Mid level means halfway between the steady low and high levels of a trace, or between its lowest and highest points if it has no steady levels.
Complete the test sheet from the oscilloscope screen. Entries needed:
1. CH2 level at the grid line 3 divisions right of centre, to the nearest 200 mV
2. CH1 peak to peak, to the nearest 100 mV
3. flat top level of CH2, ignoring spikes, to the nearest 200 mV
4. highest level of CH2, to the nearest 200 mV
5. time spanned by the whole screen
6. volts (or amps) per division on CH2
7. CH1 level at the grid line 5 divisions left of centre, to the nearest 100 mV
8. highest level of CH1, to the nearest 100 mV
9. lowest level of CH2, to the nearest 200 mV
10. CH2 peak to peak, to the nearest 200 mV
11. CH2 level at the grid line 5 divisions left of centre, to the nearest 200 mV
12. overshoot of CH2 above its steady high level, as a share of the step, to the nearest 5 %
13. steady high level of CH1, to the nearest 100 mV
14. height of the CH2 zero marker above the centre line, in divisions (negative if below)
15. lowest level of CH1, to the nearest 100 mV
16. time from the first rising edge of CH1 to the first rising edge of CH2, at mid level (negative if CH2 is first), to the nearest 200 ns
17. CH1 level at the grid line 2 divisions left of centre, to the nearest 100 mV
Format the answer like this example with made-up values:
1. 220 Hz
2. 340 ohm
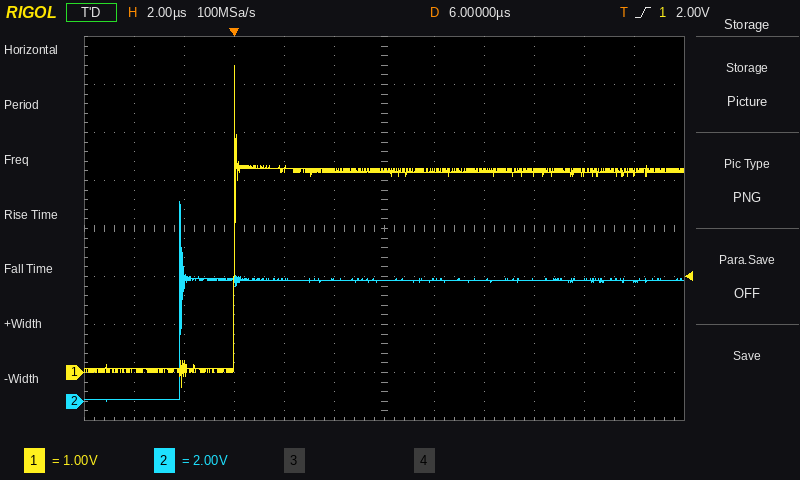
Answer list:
1. 5.0 V
2. 6.7 V
3. 5.0 V
4. 8.4 V
5. 24 µs
6. 2 V
7. 0.0 V
8. 6.4 V
9. 0.0 V
10. 8.4 V
11. 0.0 V
12. 65 %
13. 4.2 V
14. -3.6 div
15. -300 mV
16. -2.2 µs
17. 4.2 V
